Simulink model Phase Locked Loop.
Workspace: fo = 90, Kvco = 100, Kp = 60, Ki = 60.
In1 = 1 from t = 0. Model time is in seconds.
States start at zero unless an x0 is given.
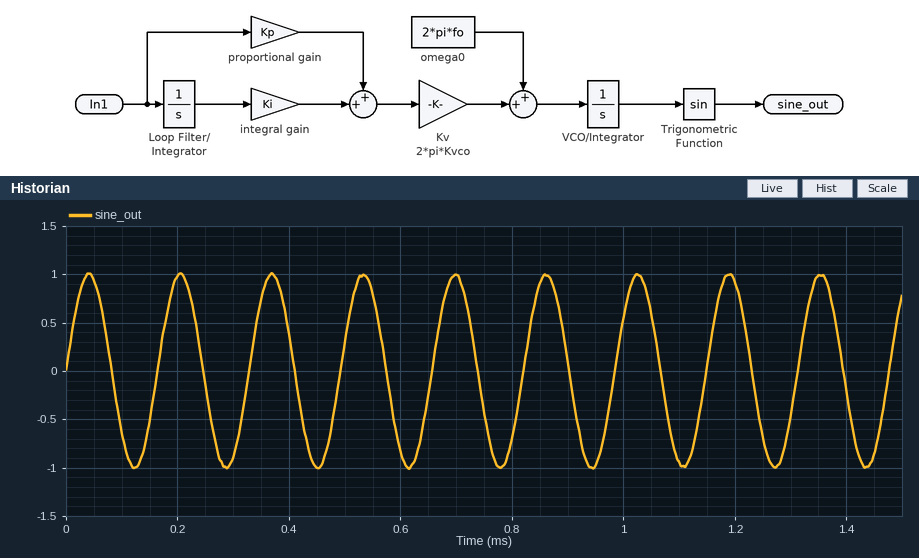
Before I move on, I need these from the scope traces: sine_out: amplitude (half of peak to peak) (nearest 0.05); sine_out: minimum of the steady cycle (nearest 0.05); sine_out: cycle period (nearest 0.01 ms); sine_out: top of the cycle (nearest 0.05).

1.00
-1.00
0.16 ms
1.00
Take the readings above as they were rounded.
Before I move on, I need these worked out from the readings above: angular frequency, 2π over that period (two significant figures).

39 rad/ms
